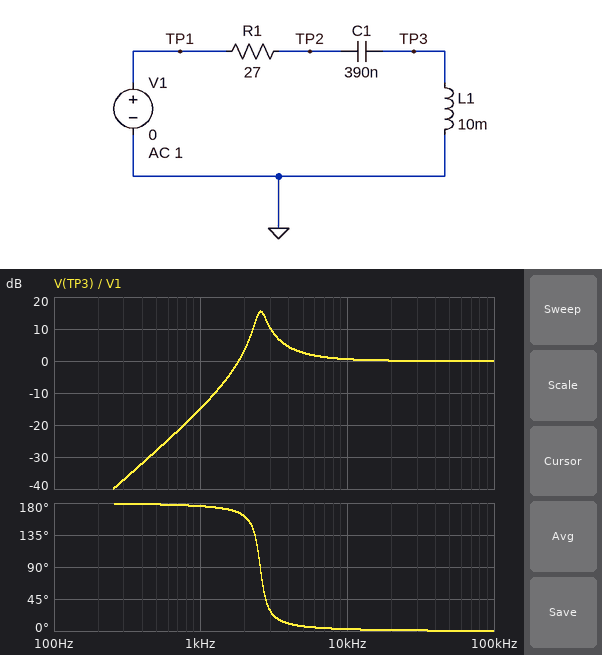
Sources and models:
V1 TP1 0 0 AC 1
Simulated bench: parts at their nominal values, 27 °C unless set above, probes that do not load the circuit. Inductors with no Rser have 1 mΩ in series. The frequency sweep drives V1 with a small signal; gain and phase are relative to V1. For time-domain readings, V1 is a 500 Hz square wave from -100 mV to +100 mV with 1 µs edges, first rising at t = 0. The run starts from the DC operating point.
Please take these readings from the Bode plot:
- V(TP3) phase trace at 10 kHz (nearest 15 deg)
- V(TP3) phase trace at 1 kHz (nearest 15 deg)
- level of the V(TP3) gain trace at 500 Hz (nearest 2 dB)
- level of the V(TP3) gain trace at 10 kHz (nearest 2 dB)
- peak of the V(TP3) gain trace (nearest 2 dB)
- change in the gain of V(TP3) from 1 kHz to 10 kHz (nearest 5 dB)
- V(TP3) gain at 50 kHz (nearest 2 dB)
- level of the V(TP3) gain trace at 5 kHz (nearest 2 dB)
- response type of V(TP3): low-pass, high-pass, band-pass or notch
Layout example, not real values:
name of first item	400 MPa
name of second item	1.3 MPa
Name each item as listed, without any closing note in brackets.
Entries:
V(TP3) phase trace at 10 kHz	0 deg
V(TP3) phase trace at 1 kHz	180 deg
level of the V(TP3) gain trace at 500 Hz	-28 dB
level of the V(TP3) gain trace at 10 kHz	0 dB
peak of the V(TP3) gain trace	16 dB
change in the gain of V(TP3) from 1 kHz to 10 kHz	15 dB
V(TP3) gain at 50 kHz	0 dB
level of the V(TP3) gain trace at 5 kHz	2 dB
response type of V(TP3): low-pass, high-pass, band-pass or notch	high-pass
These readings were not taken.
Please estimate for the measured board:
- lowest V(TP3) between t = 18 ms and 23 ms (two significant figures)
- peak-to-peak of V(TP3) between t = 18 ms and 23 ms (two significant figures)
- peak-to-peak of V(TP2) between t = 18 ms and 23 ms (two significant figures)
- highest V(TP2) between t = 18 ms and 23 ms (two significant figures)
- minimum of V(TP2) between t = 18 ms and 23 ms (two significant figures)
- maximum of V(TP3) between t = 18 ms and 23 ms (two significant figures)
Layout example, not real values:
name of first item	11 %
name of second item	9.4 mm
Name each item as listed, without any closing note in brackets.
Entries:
lowest V(TP3) between t = 18 ms and 23 ms	-260 mV
peak-to-peak of V(TP3) between t = 18 ms and 23 ms	530 mV
peak-to-peak of V(TP2) between t = 18 ms and 23 ms	260 mV
highest V(TP2) between t = 18 ms and 23 ms	130 mV
minimum of V(TP2) between t = 18 ms and 23 ms	-130 mV
maximum of V(TP3) between t = 18 ms and 23 ms	260 mV
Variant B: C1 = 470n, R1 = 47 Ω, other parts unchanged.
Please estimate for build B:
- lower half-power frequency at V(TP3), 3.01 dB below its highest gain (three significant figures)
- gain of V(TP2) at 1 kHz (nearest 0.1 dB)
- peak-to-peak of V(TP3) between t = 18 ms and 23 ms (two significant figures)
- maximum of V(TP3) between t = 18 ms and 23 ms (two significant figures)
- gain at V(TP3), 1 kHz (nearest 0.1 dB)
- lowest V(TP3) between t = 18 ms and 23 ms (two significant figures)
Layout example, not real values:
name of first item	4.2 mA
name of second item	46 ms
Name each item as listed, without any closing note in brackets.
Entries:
lower half-power frequency at V(TP3), 3.01 dB below its highest gain	2.06 kHz
gain of V(TP2) at 1 kHz	-0.1 dB
peak-to-peak of V(TP3) between t = 18 ms and 23 ms	410 mV
maximum of V(TP3) between t = 18 ms and 23 ms	210 mV
gain at V(TP3), 1 kHz	-13.0 dB
lowest V(TP3) between t = 18 ms and 23 ms	-210 mV
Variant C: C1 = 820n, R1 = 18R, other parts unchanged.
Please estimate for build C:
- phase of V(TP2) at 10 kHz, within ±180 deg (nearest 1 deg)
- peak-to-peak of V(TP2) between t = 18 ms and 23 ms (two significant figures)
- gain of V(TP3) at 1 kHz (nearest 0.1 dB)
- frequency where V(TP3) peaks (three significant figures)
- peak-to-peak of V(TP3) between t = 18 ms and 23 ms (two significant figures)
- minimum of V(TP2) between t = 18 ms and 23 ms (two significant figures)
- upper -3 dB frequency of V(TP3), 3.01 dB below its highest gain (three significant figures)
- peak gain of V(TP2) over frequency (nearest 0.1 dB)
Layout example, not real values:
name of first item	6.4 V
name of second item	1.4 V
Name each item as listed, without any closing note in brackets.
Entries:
phase of V(TP2) at 10 kHz, within ±180 deg	2 deg
peak-to-peak of V(TP2) between t = 18 ms and 23 ms	240 mV
gain of V(TP3) at 1 kHz	-6.5 dB
frequency where V(TP3) peaks	1.77 kHz
peak-to-peak of V(TP3) between t = 18 ms and 23 ms	330 mV
minimum of V(TP2) between t = 18 ms and 23 ms	-120 mV
upper -3 dB frequency of V(TP3), 3.01 dB below its highest gain	1.94 kHz
peak gain of V(TP2) over frequency	0 dB
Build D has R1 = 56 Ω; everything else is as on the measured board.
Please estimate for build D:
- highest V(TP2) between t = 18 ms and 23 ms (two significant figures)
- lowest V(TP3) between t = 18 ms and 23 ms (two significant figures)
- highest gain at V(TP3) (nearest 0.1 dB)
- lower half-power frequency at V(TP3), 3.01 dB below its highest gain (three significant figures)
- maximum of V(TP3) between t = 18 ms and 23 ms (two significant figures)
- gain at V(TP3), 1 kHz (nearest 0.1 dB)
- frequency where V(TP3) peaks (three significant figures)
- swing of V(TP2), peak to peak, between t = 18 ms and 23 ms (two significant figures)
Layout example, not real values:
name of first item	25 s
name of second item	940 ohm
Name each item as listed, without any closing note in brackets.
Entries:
highest V(TP2) between t = 18 ms and 23 ms	130 mV
lowest V(TP3) between t = 18 ms and 23 ms	-210 mV
highest gain at V(TP3)	9.3 dB
lower half-power frequency at V(TP3), 3.01 dB below its highest gain	2.25 kHz
maximum of V(TP3) between t = 18 ms and 23 ms	210 mV
gain at V(TP3), 1 kHz	-14.9 dB
frequency where V(TP3) peaks	2.63 kHz
swing of V(TP2), peak to peak, between t = 18 ms and 23 ms	270 mV
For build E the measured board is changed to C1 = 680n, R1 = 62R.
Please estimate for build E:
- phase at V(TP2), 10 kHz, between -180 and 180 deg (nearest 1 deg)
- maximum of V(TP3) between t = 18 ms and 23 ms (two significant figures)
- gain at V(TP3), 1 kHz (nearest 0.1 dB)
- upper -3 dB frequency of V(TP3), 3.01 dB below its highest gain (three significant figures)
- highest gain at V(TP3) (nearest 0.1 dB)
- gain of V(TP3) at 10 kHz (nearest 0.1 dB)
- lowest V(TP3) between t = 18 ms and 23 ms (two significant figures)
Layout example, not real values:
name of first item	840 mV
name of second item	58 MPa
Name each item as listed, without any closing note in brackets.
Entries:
phase at V(TP2), 10 kHz, between -180 and 180 deg	6 deg
maximum of V(TP3) between t = 18 ms and 23 ms	190 mV
gain at V(TP3), 1 kHz	-9.2 dB
upper -3 dB frequency of V(TP3), 3.01 dB below its highest gain	3.15 kHz
highest gain at V(TP3)	6.1 dB
gain of V(TP3) at 10 kHz	0.3 dB
lowest V(TP3) between t = 18 ms and 23 ms	-190 mV
